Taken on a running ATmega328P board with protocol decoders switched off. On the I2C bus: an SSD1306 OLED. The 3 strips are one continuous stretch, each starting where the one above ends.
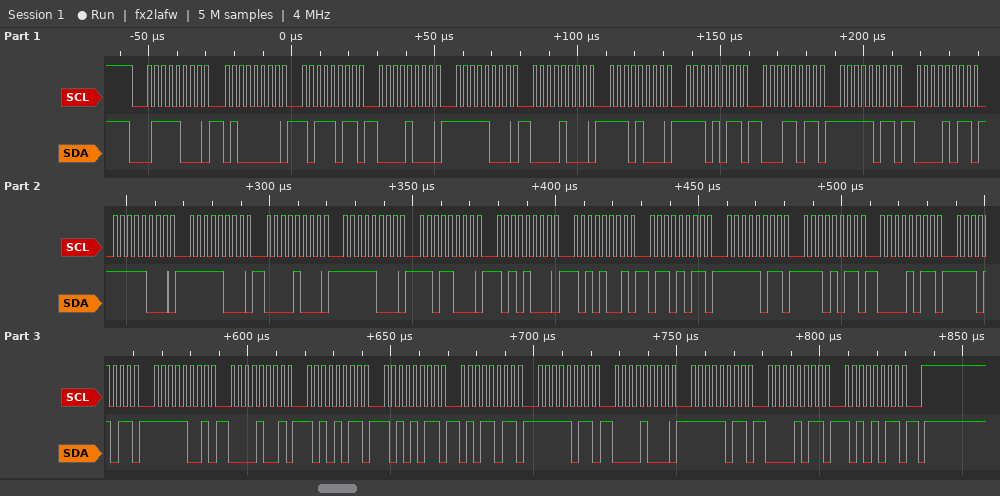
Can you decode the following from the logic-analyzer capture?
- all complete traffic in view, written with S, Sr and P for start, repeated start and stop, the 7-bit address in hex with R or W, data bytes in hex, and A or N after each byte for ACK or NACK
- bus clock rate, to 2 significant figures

S 3CW A 40 A BB A 08 A F8 A 08 A E8 A EB A 1B A FB A 0B A F8 A F8 A 08 A F8 A D8 A A8 A A9 A 6B A FB A EB A 0B A EB A F9 A 09 A AB A AB A 5B A FB A 08 A FB A 0B A AB A P
400 kHz
